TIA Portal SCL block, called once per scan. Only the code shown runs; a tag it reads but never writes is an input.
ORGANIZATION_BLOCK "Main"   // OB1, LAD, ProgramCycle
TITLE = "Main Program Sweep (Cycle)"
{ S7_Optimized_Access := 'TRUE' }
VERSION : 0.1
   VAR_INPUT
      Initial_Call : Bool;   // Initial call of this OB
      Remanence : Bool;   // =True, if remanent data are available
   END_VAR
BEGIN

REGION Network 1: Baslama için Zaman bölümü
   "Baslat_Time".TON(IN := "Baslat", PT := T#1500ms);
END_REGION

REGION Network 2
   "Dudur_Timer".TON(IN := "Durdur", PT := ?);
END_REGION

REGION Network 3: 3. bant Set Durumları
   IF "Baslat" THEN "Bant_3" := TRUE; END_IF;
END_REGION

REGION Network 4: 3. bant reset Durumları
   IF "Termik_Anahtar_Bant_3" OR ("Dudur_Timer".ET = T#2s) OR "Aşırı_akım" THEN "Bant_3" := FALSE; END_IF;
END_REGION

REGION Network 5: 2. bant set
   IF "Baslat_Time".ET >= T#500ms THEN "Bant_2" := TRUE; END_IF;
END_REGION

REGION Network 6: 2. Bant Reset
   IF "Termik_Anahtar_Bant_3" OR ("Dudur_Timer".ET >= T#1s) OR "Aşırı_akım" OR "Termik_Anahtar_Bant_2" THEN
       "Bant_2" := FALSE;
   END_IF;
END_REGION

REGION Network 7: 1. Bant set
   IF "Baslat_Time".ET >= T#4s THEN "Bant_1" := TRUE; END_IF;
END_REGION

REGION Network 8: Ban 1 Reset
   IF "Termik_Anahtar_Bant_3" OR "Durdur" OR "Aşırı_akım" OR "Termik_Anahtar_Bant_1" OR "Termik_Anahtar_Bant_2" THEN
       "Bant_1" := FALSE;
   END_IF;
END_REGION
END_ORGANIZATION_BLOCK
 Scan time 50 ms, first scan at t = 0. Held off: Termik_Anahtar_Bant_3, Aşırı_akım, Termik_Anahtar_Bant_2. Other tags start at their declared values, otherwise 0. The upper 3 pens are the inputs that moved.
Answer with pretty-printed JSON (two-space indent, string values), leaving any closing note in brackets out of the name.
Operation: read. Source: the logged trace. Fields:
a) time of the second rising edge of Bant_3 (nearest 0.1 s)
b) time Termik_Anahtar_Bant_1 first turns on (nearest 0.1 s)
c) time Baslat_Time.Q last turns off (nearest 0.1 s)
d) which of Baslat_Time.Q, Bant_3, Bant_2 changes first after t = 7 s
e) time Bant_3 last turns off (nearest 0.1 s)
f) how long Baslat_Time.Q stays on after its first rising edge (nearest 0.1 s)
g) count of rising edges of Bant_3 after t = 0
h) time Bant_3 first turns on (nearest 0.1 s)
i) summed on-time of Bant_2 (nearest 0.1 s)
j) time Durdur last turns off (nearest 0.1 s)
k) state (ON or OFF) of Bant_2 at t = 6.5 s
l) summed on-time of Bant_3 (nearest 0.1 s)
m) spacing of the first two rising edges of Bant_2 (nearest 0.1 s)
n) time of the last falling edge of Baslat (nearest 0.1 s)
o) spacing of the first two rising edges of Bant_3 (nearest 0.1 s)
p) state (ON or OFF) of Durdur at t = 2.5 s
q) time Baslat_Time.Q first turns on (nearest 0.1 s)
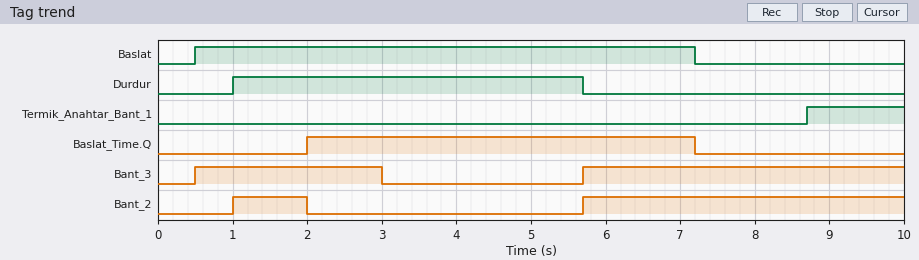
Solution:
{
  "time of the second rising edge of Bant_3": "5.7 s",
  "time Termik_Anahtar_Bant_1 first turns on": "8.7 s",
  "time Baslat_Time.Q last turns off": "7.2 s",
  "which of Baslat_Time.Q, Bant_3, Bant_2 changes first after t = 7 s": "Baslat_Time.Q",
  "time Bant_3 last turns off": "3.0 s",
  "how long Baslat_Time.Q stays on after its first rising edge": "5.2 s",
  "count of rising edges of Bant_3 after t = 0": "2",
  "time Bant_3 first turns on": "0.5 s",
  "summed on-time of Bant_2": "5.3 s",
  "time Durdur last turns off": "5.7 s",
  "state (ON or OFF) of Bant_2 at t = 6.5 s": "ON",
  "summed on-time of Bant_3": "6.8 s",
  "spacing of the first two rising edges of Bant_2": "4.7 s",
  "time of the last falling edge of Baslat": "7.2 s",
  "spacing of the first two rising edges of Bant_3": "5.2 s",
  "state (ON or OFF) of Durdur at t = 2.5 s": "ON",
  "time Baslat_Time.Q first turns on": "2.0 s"
}
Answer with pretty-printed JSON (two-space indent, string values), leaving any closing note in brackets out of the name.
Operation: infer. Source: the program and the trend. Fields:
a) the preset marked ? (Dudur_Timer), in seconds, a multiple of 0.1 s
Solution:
{
  "the preset marked ? (Dudur_Timer), in seconds, a multiple of 0.1 s": "2.0 s"
}
